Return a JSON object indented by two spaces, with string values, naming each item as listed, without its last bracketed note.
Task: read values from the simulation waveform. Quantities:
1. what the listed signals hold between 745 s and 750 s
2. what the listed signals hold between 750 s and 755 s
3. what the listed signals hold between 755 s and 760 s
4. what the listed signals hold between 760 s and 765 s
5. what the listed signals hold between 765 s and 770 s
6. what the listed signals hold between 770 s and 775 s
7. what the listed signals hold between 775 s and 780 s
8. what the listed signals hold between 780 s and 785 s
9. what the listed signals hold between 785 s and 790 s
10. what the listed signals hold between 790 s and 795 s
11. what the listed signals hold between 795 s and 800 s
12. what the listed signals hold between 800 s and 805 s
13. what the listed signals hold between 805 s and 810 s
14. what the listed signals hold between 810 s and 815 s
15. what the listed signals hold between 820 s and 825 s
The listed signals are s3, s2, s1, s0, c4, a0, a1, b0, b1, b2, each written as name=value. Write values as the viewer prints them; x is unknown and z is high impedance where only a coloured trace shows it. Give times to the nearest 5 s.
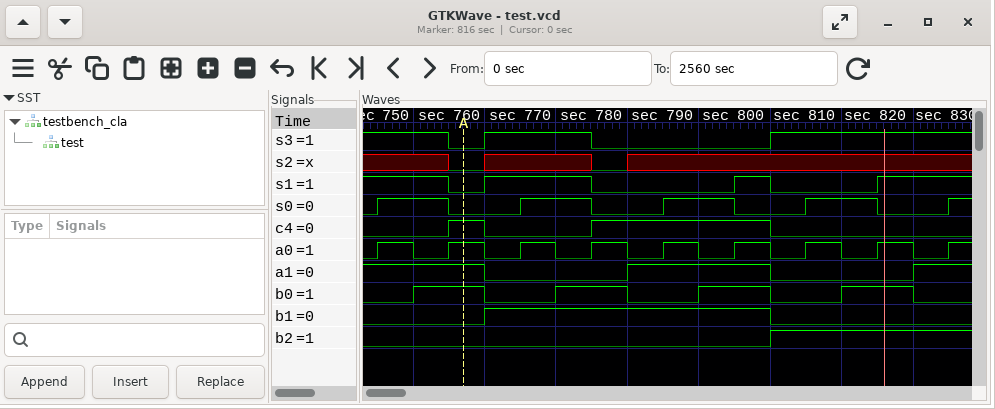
{
  "what the listed signals hold between 745 s and 750 s": "s3=1, s2=x, s1=1, s0=1, c4=0, a0=1, a1=1, b0=0, b1=0, b2=0",
  "what the listed signals hold between 750 s and 755 s": "s3=1, s2=x, s1=1, s0=1, c4=0, a0=0, a1=1, b0=1, b1=0, b2=0",
  "what the listed signals hold between 755 s and 760 s": "s3=0, s2=0, s1=0, s0=0, c4=1, a0=1, a1=1, b0=1, b1=0, b2=0",
  "what the listed signals hold between 760 s and 765 s": "s3=1, s2=x, s1=1, s0=0, c4=0, a0=0, a1=0, b0=0, b1=1, b2=0",
  "what the listed signals hold between 765 s and 770 s": "s3=1, s2=x, s1=1, s0=1, c4=0, a0=1, a1=0, b0=0, b1=1, b2=0",
  "what the listed signals hold between 770 s and 775 s": "s3=1, s2=x, s1=1, s0=1, c4=0, a0=0, a1=0, b0=1, b1=1, b2=0",
  "what the listed signals hold between 775 s and 780 s": "s3=0, s2=0, s1=0, s0=0, c4=1, a0=1, a1=0, b0=1, b1=1, b2=0",
  "what the listed signals hold between 780 s and 785 s": "s3=0, s2=x, s1=0, s0=0, c4=1, a0=0, a1=1, b0=0, b1=1, b2=0",
  "what the listed signals hold between 785 s and 790 s": "s3=0, s2=x, s1=0, s0=1, c4=1, a0=1, a1=1, b0=0, b1=1, b2=0",
  "what the listed signals hold between 790 s and 795 s": "s3=0, s2=x, s1=0, s0=1, c4=1, a0=0, a1=1, b0=1, b1=1, b2=0",
  "what the listed signals hold between 795 s and 800 s": "s3=0, s2=x, s1=1, s0=0, c4=1, a0=1, a1=1, b0=1, b1=1, b2=0",
  "what the listed signals hold between 800 s and 805 s": "s3=1, s2=x, s1=0, s0=0, c4=0, a0=0, a1=0, b0=0, b1=0, b2=1",
  "what the listed signals hold between 805 s and 810 s": "s3=1, s2=x, s1=0, s0=1, c4=0, a0=1, a1=0, b0=0, b1=0, b2=1",
  "what the listed signals hold between 810 s and 815 s": "s3=1, s2=x, s1=0, s0=1, c4=0, a0=0, a1=0, b0=1, b1=0, b2=1",
  "what the listed signals hold between 820 s and 825 s": "s3=1, s2=x, s1=1, s0=0, c4=0, a0=0, a1=1, b0=0, b1=0, b2=1"
}
